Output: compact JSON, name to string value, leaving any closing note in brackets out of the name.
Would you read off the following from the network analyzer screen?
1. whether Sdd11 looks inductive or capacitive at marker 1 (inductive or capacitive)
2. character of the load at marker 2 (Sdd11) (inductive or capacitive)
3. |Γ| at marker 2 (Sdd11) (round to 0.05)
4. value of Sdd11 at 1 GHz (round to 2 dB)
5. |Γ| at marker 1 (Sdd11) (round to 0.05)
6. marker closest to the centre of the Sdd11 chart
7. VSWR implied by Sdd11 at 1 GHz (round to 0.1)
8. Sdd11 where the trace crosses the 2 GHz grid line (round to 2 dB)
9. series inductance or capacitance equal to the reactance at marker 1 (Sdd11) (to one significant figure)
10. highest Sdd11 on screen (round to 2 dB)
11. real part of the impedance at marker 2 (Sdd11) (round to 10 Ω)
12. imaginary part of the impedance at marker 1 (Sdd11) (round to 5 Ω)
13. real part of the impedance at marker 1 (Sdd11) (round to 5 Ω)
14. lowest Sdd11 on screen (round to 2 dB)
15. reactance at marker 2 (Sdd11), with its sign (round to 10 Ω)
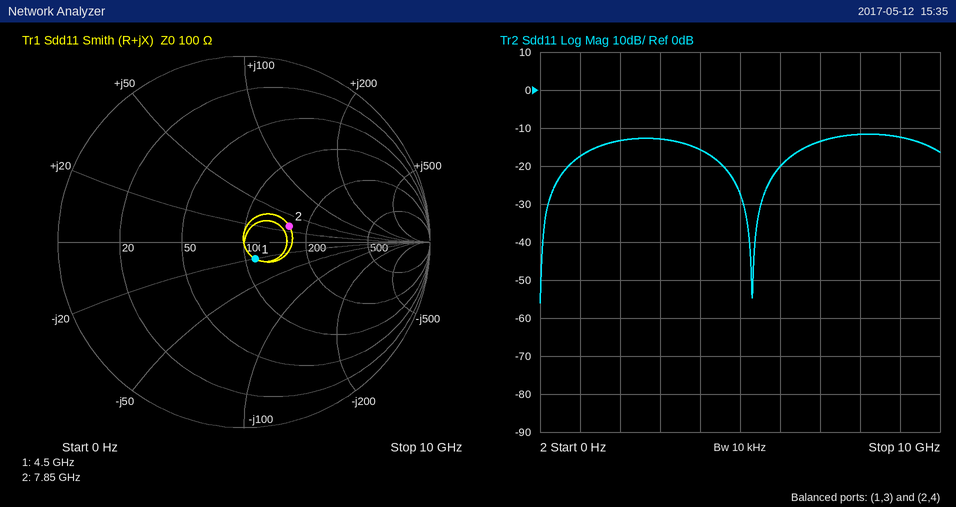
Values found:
{"whether Sdd11 looks inductive or capacitive at marker 1": "capacitive", "character of the load at marker 2 (Sdd11)": "inductive", "|Γ| at marker 2 (Sdd11)": "0.25", "value of Sdd11 at 1 GHz": "-18 dB", "|Γ| at marker 1 (Sdd11)": "0.10", "marker closest to the centre of the Sdd11 chart": "marker 1", "VSWR implied by Sdd11 at 1 GHz": "1.3", "Sdd11 where the trace crosses the 2 GHz grid line": "-14 dB", "series inductance or capacitance equal to the reactance at marker 1 (Sdd11)": "2 pF", "highest Sdd11 on screen": "-12 dB", "real part of the impedance at marker 2 (Sdd11)": "160 Ω", "imaginary part of the impedance at marker 1 (Sdd11)": "-20 Ω", "real part of the impedance at marker 1 (Sdd11)": "110 Ω", "lowest Sdd11 on screen": "-56 dB", "reactance at marker 2 (Sdd11), with its sign": "+30 Ω"}
